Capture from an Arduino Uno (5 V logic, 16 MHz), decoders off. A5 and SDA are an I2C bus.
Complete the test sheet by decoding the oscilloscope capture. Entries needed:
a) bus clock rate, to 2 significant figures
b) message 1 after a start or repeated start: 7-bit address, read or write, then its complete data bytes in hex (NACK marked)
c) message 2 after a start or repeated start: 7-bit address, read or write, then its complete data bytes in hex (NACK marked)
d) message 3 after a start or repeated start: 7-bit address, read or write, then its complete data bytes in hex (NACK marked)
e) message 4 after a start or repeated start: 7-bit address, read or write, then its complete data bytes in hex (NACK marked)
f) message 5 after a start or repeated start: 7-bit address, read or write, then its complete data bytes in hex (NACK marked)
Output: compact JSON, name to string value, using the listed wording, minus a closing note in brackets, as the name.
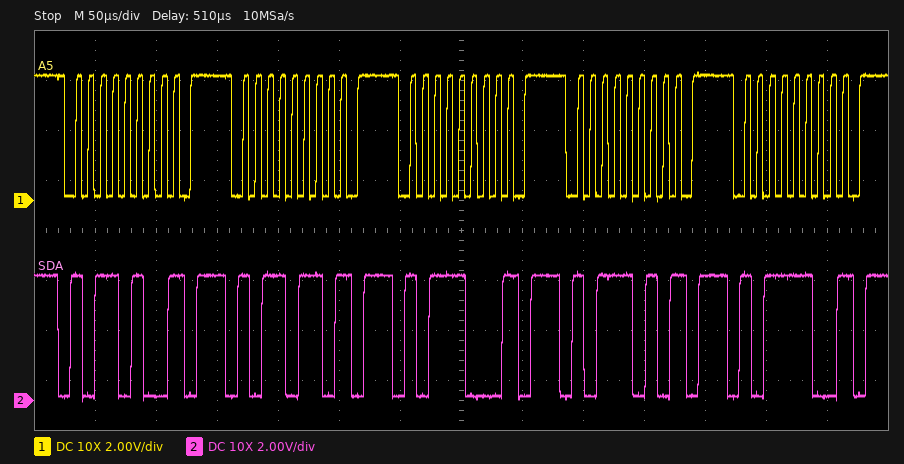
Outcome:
{"bus clock rate, to 2 significant figures": "100 kHz", "message 1 after a start or repeated start: 7-bit address, read or write, then its complete data bytes in hex": "0x5A write NACK", "message 2 after a start or repeated start: 7-bit address, read or write, then its complete data bytes in hex": "0x5B write NACK", "message 3 after a start or repeated start: 7-bit address, read or write, then its complete data bytes in hex": "0x5C write NACK", "message 4 after a start or repeated start: 7-bit address, read or write, then its complete data bytes in hex": "0x5D write NACK", "message 5 after a start or repeated start: 7-bit address, read or write, then its complete data bytes in hex": "0x5E write NACK"}
